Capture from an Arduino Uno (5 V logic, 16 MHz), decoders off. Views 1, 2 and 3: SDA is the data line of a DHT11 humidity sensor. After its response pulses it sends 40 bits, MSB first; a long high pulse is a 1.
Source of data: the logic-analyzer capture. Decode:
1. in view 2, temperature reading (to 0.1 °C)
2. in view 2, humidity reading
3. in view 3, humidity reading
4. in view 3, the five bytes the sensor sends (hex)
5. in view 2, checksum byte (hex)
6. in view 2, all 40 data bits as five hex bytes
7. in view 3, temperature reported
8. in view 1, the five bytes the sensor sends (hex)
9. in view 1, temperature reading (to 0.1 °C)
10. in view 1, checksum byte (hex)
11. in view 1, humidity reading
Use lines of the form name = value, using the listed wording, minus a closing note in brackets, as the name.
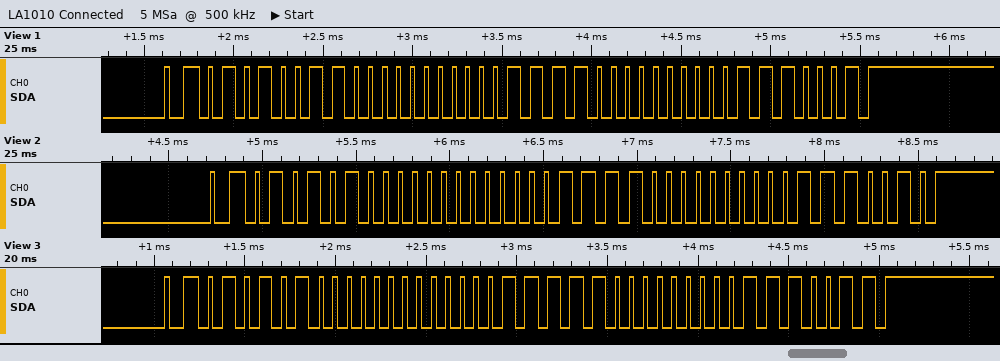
in view 2, temperature reading = 30.0 °C
in view 2, humidity reading = 84 %
in view 3, humidity reading = 84 %
in view 3, the five bytes the sensor sends = 54 00 1F 00 73
in view 2, checksum byte = 0x72
in view 2, all 40 data bits as five hex bytes = 54 00 1E 00 72
in view 3, temperature reported = 31.0 °C
in view 1, the five bytes the sensor sends = 53 00 1E 00 71
in view 1, temperature reading = 30.0 °C
in view 1, checksum byte = 0x71
in view 1, humidity reading = 83 %
